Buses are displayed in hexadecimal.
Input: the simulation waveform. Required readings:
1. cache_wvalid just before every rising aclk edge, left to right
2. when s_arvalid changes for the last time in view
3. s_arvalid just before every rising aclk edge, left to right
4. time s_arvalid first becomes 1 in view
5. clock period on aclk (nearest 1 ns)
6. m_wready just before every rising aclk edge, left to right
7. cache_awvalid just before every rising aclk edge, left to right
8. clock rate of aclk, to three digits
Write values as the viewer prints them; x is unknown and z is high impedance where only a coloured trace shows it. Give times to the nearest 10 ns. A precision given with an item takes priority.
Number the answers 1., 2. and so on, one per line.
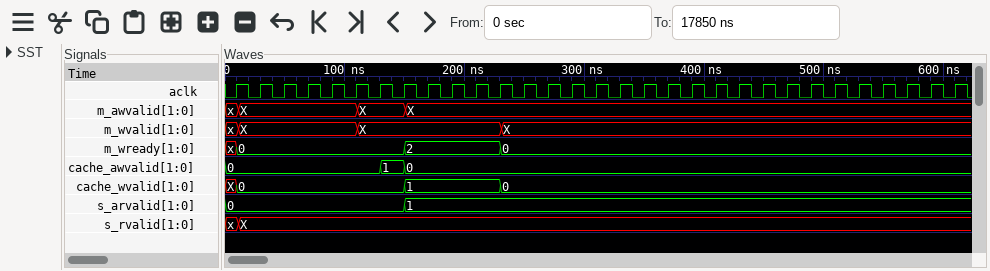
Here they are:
1. X, 0, 0, 0, 0, 0, 0, 0, 1, 1, 1, 1, 0, 0, 0, 0, 0, 0, 0, 0, 0, 0, 0, 0, 0, 0, 0, 0, 0, 0, 0
2. 150 ns
3. 0, 0, 0, 0, 0, 0, 0, 0, 1, 1, 1, 1, 1, 1, 1, 1, 1, 1, 1, 1, 1, 1, 1, 1, 1, 1, 1, 1, 1, 1, 1
4. 150 ns
5. 20 ns
6. x, 0, 0, 0, 0, 0, 0, 0, 2, 2, 2, 2, 0, 0, 0, 0, 0, 0, 0, 0, 0, 0, 0, 0, 0, 0, 0, 0, 0, 0, 0
7. 0, 0, 0, 0, 0, 0, 0, 1, 0, 0, 0, 0, 0, 0, 0, 0, 0, 0, 0, 0, 0, 0, 0, 0, 0, 0, 0, 0, 0, 0, 0
8. 50.0 MHz
